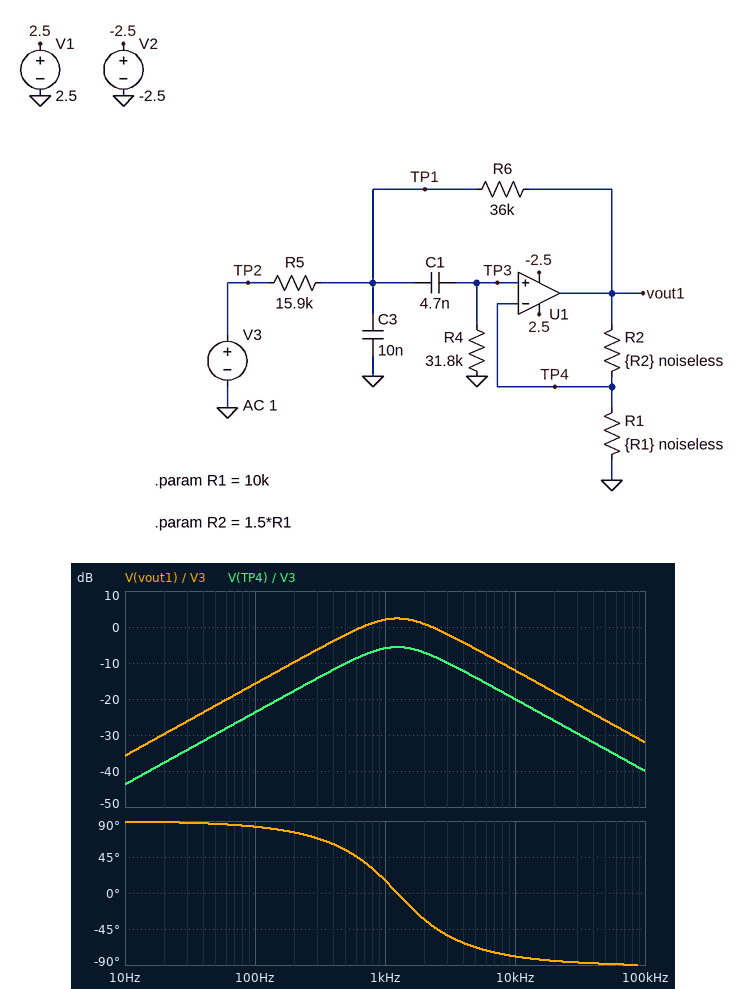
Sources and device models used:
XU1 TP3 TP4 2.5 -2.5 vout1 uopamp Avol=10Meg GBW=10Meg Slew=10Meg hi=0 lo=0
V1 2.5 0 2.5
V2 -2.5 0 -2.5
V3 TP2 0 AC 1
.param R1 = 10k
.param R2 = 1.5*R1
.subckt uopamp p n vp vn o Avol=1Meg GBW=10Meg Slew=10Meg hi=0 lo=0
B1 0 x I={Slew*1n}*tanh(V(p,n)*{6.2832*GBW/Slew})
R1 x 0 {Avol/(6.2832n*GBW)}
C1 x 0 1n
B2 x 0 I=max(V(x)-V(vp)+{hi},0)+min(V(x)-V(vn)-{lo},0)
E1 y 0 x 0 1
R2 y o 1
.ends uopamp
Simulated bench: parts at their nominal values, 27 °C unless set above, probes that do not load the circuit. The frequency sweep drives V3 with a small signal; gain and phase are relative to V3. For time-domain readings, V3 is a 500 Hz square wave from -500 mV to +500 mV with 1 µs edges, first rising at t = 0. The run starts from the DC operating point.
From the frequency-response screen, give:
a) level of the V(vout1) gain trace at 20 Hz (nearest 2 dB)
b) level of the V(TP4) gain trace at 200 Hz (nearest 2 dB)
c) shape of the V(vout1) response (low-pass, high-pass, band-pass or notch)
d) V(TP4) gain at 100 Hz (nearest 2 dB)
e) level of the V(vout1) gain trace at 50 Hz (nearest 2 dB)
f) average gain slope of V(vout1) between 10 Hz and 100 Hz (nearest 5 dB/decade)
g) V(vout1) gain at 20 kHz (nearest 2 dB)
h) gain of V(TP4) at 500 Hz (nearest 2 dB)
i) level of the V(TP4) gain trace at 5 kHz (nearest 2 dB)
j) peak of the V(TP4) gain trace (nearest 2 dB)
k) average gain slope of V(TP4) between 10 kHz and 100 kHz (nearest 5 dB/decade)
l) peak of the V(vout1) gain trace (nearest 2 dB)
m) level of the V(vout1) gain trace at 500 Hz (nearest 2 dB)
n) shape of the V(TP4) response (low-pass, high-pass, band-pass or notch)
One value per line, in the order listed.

-30 dB
-18 dB
band-pass
-24 dB
-22 dB
20 dB/decade
-18 dB
-10 dB
-14 dB
-6 dB
-20 dB/decade
2 dB
-2 dB
band-pass
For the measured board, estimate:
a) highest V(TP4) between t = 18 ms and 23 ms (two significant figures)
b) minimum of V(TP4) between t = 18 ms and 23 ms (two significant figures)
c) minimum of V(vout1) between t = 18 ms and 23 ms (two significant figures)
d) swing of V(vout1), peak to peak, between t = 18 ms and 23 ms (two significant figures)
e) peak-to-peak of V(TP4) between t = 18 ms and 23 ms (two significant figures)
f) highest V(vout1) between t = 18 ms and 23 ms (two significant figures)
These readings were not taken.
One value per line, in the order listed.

350 mV
-350 mV
-880 mV
1.8 V
700 mV
880 mV
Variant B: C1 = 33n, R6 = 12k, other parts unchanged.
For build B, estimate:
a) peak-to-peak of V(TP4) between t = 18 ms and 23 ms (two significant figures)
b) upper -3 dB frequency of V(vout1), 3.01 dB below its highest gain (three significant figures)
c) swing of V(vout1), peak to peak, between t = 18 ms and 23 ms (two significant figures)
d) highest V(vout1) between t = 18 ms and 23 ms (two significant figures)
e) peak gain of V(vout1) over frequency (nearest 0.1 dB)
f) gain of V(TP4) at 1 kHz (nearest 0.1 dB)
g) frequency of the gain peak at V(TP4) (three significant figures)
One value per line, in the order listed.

2.0 V
785 Hz
5.0 V
2.5 V
17.4 dB
2.7 dB
594 Hz
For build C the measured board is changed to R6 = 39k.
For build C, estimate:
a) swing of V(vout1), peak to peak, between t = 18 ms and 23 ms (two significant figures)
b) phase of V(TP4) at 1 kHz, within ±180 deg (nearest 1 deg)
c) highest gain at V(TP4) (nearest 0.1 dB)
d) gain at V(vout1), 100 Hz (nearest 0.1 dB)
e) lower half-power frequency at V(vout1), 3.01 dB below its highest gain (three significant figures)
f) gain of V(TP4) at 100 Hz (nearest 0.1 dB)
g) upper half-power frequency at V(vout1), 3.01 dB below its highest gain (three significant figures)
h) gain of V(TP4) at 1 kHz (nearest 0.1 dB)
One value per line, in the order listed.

1.7 V
14 deg
-5.8 dB
-15.6 dB
590 Hz
-23.5 dB
2.54 kHz
-6.1 dB
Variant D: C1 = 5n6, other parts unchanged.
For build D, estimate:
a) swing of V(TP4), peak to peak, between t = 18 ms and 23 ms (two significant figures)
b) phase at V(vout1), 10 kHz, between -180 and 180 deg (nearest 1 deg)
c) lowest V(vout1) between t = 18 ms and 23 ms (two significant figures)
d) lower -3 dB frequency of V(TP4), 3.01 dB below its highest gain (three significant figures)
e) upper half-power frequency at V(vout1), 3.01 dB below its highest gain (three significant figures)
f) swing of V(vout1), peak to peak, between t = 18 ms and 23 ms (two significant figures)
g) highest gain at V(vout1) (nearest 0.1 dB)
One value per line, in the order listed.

770 mV
-80 deg
-970 mV
562 Hz
2.29 kHz
1.9 V
3.2 dB
